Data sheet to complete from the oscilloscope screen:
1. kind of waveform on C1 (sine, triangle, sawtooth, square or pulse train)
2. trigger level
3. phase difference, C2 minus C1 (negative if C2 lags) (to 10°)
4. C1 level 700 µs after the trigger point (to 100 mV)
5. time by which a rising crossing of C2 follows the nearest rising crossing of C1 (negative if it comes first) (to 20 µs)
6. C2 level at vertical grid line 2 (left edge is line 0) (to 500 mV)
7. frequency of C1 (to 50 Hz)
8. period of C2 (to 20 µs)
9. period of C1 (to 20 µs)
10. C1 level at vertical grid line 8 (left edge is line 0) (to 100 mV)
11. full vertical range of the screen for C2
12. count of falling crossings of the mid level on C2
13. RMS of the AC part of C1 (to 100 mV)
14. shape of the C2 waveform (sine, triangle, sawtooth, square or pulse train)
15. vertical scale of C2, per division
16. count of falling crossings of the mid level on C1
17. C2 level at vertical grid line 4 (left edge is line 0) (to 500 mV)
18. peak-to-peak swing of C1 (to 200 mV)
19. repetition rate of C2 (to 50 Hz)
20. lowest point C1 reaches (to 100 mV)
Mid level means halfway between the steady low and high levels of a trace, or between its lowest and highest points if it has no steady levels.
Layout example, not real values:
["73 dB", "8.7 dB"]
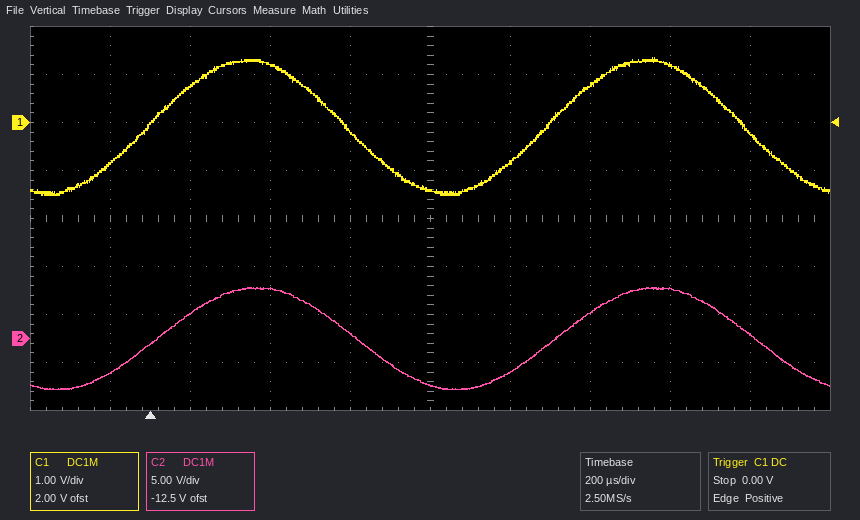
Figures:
["sine", "0.00 V", "-10°", "-1.4 V", "+20 µs", "2.5 V", "1.00 kHz", "1.00 ms", "1.00 ms", "1.2 V", "40 V", "2", "1.0 V", "sine", "5 V", "2", "500 mV", "2.8 V", "1.00 kHz", "-1.5 V"]
